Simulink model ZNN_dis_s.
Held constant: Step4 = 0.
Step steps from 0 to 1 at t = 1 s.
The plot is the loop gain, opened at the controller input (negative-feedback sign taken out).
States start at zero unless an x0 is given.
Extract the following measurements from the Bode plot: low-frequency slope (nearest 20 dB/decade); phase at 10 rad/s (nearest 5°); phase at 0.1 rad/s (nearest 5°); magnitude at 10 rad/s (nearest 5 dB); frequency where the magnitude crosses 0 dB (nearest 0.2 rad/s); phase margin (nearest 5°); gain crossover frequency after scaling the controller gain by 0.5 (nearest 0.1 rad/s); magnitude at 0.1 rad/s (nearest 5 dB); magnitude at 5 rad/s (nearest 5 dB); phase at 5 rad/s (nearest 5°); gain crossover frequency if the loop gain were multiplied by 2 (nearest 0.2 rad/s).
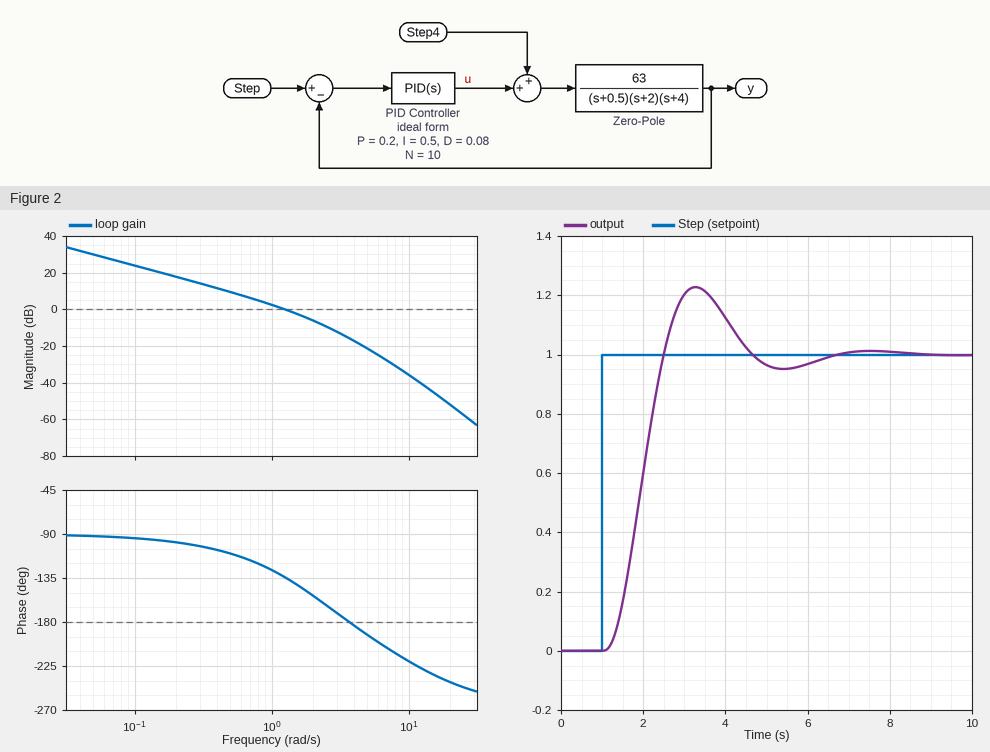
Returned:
-20 dB/decade
-220°
-95°
-35 dB
1.2 rad/s
45°
0.7 rad/s
25 dB
-20 dB
-195°
2.0 rad/s
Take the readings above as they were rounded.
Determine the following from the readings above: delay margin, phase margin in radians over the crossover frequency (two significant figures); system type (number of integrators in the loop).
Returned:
0.65 s
1
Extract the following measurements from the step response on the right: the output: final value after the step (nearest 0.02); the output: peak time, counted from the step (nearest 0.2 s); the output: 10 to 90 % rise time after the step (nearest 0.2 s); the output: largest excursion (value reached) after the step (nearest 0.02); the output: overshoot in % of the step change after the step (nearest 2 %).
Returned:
1.00
2.2 s
1.0 s
1.22
22 %
